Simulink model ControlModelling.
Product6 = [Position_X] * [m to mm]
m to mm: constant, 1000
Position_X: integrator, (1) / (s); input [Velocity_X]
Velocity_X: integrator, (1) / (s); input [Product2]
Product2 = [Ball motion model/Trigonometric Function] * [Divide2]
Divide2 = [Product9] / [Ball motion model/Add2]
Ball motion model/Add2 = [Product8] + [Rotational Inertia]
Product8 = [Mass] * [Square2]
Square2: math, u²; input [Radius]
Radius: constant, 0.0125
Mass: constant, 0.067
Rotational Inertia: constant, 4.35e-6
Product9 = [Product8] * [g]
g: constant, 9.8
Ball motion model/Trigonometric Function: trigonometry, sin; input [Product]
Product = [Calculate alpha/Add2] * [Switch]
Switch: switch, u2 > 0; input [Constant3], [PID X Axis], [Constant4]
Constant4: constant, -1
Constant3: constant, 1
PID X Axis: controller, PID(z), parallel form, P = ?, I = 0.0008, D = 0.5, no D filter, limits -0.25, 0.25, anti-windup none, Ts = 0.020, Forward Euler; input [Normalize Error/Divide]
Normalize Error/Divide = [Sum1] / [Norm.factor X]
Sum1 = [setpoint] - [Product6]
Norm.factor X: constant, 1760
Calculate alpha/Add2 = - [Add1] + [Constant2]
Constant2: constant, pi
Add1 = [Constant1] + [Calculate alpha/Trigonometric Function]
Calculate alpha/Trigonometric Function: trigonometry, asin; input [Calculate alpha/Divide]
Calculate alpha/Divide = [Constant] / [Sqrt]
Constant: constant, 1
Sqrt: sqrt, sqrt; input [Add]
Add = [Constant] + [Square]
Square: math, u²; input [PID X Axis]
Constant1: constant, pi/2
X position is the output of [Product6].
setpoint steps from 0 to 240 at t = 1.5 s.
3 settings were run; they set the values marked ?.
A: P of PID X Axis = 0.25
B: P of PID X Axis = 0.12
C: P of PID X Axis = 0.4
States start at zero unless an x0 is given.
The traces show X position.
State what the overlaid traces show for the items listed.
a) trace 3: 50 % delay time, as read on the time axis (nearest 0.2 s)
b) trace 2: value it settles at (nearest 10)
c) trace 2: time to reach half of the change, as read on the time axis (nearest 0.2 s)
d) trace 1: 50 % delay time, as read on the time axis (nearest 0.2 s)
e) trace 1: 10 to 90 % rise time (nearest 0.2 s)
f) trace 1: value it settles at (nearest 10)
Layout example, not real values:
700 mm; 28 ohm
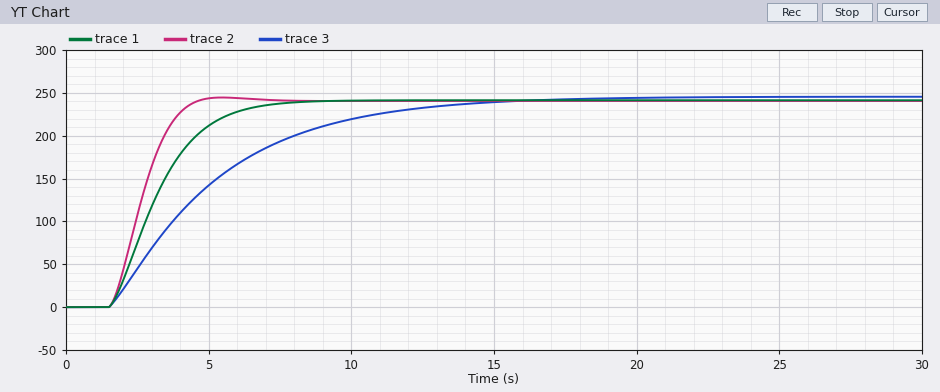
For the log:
4.4 s; 240; 2.6 s; 3.0 s; 3.4 s; 240
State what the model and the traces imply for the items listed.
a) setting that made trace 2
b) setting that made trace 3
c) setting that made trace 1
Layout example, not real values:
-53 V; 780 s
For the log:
C; B; A
